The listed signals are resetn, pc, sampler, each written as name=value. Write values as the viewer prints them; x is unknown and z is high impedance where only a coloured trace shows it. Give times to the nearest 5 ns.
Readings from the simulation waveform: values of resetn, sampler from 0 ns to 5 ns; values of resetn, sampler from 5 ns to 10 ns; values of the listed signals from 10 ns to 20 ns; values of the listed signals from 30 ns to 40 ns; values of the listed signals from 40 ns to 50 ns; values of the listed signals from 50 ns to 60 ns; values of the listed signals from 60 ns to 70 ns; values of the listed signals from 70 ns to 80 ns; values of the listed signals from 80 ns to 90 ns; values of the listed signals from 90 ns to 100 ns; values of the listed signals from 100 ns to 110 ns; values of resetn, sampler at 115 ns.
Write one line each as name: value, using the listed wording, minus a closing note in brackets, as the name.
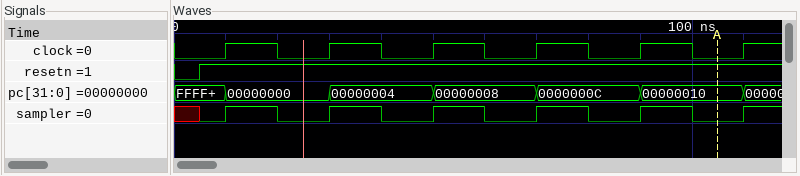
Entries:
values of resetn, sampler from 0 ns to 5 ns: resetn=0, sampler=x
values of resetn, sampler from 5 ns to 10 ns: resetn=1, sampler=0
values of the listed signals from 10 ns to 20 ns: resetn=1, pc=00000000, sampler=1
values of the listed signals from 30 ns to 40 ns: resetn=1, pc=00000004, sampler=1
values of the listed signals from 40 ns to 50 ns: resetn=1, pc=00000004, sampler=0
values of the listed signals from 50 ns to 60 ns: resetn=1, pc=00000008, sampler=1
values of the listed signals from 60 ns to 70 ns: resetn=1, pc=00000008, sampler=0
values of the listed signals from 70 ns to 80 ns: resetn=1, pc=0000000C, sampler=1
values of the listed signals from 80 ns to 90 ns: resetn=1, pc=0000000C, sampler=0
values of the listed signals from 90 ns to 100 ns: resetn=1, pc=00000010, sampler=1
values of the listed signals from 100 ns to 110 ns: resetn=1, pc=00000010, sampler=0
values of resetn, sampler at 115 ns: resetn=1, sampler=1
